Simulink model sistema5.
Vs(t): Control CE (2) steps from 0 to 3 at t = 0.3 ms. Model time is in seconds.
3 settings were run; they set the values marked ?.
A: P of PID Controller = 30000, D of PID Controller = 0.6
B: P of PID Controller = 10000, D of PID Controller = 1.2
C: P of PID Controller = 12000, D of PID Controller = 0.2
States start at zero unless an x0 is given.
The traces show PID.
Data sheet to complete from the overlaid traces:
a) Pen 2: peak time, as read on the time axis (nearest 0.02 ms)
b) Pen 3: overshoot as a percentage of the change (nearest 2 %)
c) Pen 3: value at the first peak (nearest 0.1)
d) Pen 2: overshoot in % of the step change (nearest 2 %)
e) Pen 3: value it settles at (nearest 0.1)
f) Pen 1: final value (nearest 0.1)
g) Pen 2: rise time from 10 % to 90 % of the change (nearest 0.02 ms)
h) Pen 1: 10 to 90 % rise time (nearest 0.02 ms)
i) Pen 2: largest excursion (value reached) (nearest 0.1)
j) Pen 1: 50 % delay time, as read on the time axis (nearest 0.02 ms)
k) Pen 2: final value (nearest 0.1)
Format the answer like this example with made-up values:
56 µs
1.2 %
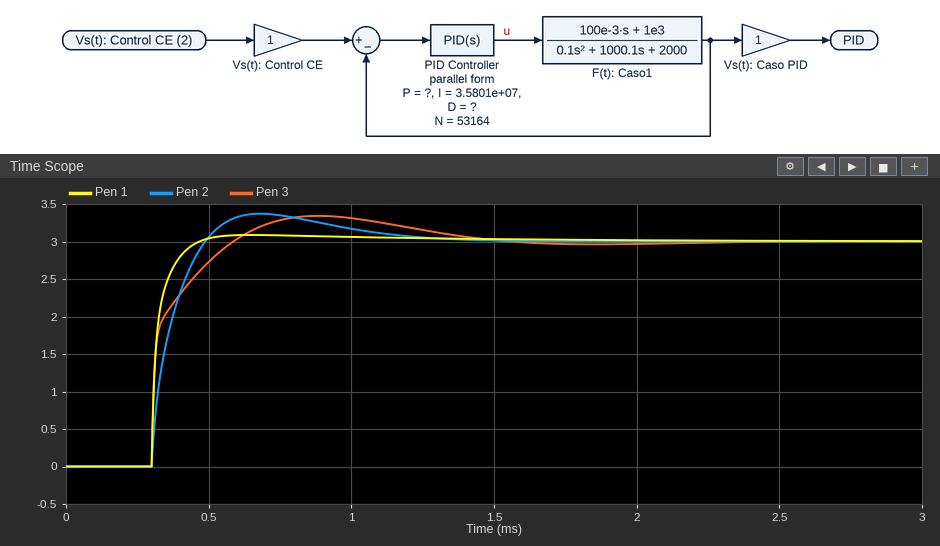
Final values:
0.68 ms
12 %
3.3
12 %
3.0
3.0
0.14 ms
0.08 ms
3.4
0.32 ms
3.0
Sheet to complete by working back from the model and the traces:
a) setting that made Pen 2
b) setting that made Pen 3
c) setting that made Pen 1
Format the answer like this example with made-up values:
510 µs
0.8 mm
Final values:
C
B
A
